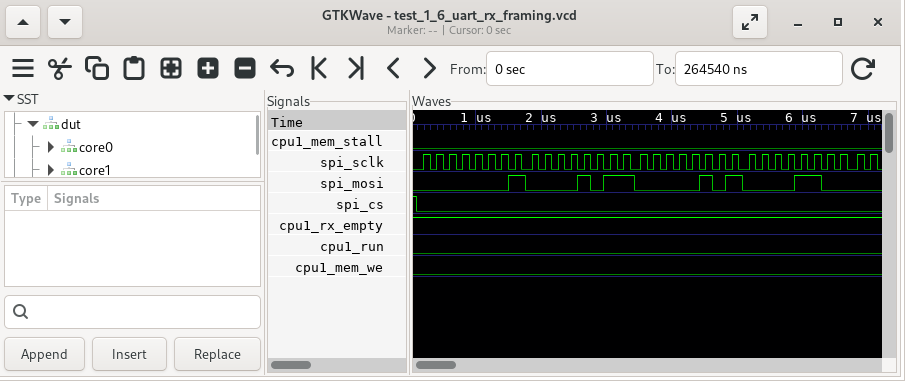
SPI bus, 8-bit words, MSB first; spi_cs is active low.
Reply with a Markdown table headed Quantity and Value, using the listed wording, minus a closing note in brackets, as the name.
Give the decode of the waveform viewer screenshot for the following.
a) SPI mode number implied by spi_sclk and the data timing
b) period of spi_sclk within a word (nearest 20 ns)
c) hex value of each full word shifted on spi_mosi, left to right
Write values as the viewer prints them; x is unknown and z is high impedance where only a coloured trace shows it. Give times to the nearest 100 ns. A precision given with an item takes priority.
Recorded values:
| Quantity | Value |
|---|---|
| SPI mode number implied by spi_sclk and the data timing | 0 |
| period of spi_sclk within a word | 200 ns |
| hex value of each full word shifted on spi_mosi, left to right | 01, 0B, 05, 0C |
